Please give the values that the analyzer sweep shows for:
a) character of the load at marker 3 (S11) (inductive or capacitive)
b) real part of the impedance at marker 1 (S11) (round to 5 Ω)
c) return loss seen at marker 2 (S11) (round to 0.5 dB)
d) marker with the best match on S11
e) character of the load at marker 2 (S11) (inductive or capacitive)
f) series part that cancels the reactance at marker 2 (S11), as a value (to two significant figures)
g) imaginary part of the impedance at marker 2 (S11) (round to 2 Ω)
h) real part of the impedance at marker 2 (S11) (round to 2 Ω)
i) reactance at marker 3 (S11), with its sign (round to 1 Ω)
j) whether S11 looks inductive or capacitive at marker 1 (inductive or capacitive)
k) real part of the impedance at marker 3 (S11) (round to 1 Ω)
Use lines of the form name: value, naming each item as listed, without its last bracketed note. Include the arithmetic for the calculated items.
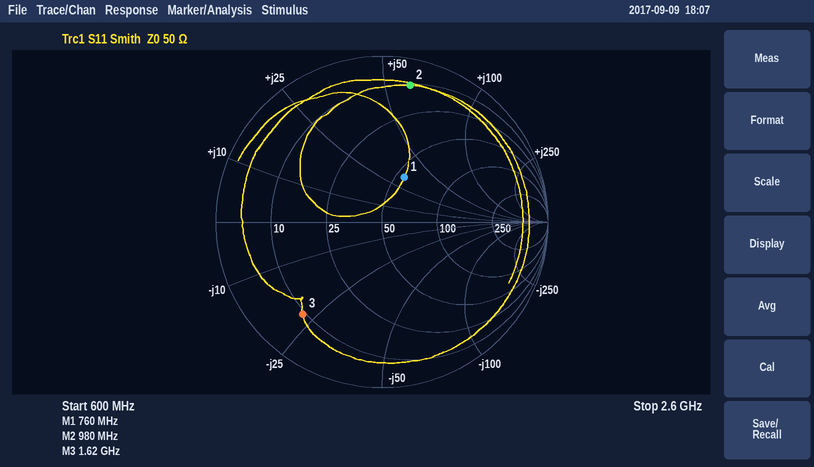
character of the load at marker 3 (S11): capacitive
real part of the impedance at marker 1 (S11): 55 Ω
return loss seen at marker 2 (S11): 1.5 dB
marker with the best match on S11: marker 1
character of the load at marker 2 (S11): inductive
series part that cancels the reactance at marker 2 (S11), as a value: C = 1/(2π × 980 MHz × 60 Ω) ≈ 2.7 pF
imaginary part of the impedance at marker 2 (S11): +60 Ω
real part of the impedance at marker 2 (S11): 10 Ω
reactance at marker 3 (S11), with its sign: -22 Ω
whether S11 looks inductive or capacitive at marker 1: inductive
real part of the impedance at marker 3 (S11): 9 Ω
